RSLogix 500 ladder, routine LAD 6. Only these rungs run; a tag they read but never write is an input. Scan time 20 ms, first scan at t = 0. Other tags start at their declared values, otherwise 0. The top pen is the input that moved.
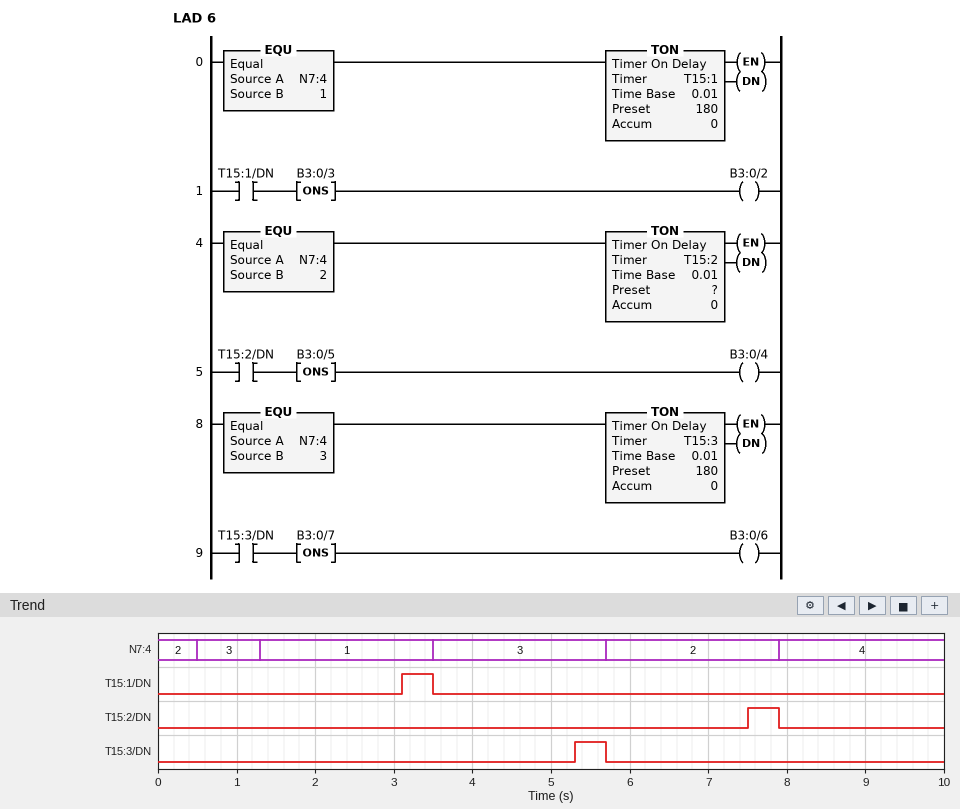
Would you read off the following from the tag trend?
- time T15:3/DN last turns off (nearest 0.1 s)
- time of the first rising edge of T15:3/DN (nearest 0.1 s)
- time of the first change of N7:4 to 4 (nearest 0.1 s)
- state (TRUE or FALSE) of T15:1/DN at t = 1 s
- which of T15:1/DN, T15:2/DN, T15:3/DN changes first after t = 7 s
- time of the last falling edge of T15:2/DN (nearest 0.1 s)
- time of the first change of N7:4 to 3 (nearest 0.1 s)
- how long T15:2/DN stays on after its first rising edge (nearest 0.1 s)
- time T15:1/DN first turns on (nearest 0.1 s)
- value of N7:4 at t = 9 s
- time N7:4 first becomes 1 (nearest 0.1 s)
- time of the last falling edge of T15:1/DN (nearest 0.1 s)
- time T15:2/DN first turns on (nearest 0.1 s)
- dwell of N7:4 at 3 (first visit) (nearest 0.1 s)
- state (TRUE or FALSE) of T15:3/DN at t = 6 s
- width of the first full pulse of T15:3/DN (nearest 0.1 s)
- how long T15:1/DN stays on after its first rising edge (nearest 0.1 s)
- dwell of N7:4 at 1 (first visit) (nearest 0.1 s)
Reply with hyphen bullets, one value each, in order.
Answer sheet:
- 5.7 s
- 5.3 s
- 7.9 s
- FALSE
- T15:2/DN
- 7.9 s
- 0.5 s
- 0.4 s
- 3.1 s
- 4
- 1.3 s
- 3.5 s
- 7.5 s
- 0.8 s
- FALSE
- 0.4 s
- 0.4 s
- 2.2 s
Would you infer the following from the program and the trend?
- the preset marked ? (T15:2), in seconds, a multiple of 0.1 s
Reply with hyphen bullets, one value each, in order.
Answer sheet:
- 1.8 s
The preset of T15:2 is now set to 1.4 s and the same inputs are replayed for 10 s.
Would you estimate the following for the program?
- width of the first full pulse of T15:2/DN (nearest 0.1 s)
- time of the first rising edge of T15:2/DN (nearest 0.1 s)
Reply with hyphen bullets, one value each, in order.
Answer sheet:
- 0.8 s
- 7.1 s
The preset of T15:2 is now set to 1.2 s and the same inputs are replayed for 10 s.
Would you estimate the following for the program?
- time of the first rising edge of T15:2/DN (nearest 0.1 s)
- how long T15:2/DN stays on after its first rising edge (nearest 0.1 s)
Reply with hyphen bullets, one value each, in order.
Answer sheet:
- 6.9 s
- 1.0 s
